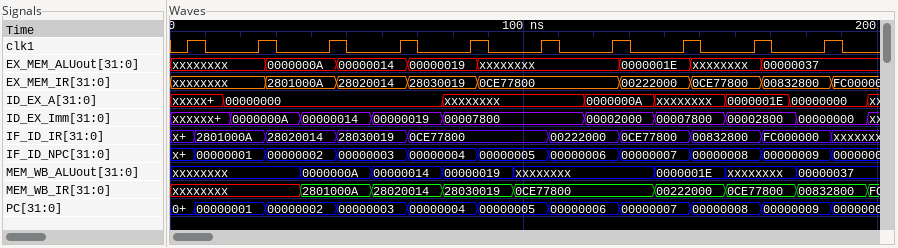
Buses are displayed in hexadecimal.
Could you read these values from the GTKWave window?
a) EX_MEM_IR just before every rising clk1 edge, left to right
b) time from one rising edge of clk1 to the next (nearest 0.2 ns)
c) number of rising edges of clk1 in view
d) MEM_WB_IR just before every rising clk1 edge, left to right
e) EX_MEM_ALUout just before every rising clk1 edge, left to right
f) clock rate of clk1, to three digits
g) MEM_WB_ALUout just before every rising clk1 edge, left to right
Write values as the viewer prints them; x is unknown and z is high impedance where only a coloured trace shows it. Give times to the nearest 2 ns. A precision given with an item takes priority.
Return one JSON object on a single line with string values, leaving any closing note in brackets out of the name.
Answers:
{"EX_MEM_IR just before every rising clk1 edge, left to right": "xxxxxxxx, xxxxxxxx, 2801000A, 28020014, 28030019, 0CE77800, 0CE77800, 00222000, 0CE77800, 00832800", "time from one rising edge of clk1 to the next": "20 ns", "number of rising edges of clk1 in view": "10", "MEM_WB_IR just before every rising clk1 edge, left to right": "xxxxxxxx, xxxxxxxx, 2801000A, 28020014, 28030019, 0CE77800, 0CE77800, 00222000, 0CE77800, 00832800", "EX_MEM_ALUout just before every rising clk1 edge, left to right": "xxxxxxxx, xxxxxxxx, 0000000A, 00000014, 00000019, xxxxxxxx, xxxxxxxx, 0000001E, xxxxxxxx, 00000037", "clock rate of clk1, to three digits": "50.0 MHz", "MEM_WB_ALUout just before every rising clk1 edge, left to right": "xxxxxxxx, xxxxxxxx, 0000000A, 00000014, 00000019, xxxxxxxx, xxxxxxxx, 0000001E, xxxxxxxx, 00000037"}
